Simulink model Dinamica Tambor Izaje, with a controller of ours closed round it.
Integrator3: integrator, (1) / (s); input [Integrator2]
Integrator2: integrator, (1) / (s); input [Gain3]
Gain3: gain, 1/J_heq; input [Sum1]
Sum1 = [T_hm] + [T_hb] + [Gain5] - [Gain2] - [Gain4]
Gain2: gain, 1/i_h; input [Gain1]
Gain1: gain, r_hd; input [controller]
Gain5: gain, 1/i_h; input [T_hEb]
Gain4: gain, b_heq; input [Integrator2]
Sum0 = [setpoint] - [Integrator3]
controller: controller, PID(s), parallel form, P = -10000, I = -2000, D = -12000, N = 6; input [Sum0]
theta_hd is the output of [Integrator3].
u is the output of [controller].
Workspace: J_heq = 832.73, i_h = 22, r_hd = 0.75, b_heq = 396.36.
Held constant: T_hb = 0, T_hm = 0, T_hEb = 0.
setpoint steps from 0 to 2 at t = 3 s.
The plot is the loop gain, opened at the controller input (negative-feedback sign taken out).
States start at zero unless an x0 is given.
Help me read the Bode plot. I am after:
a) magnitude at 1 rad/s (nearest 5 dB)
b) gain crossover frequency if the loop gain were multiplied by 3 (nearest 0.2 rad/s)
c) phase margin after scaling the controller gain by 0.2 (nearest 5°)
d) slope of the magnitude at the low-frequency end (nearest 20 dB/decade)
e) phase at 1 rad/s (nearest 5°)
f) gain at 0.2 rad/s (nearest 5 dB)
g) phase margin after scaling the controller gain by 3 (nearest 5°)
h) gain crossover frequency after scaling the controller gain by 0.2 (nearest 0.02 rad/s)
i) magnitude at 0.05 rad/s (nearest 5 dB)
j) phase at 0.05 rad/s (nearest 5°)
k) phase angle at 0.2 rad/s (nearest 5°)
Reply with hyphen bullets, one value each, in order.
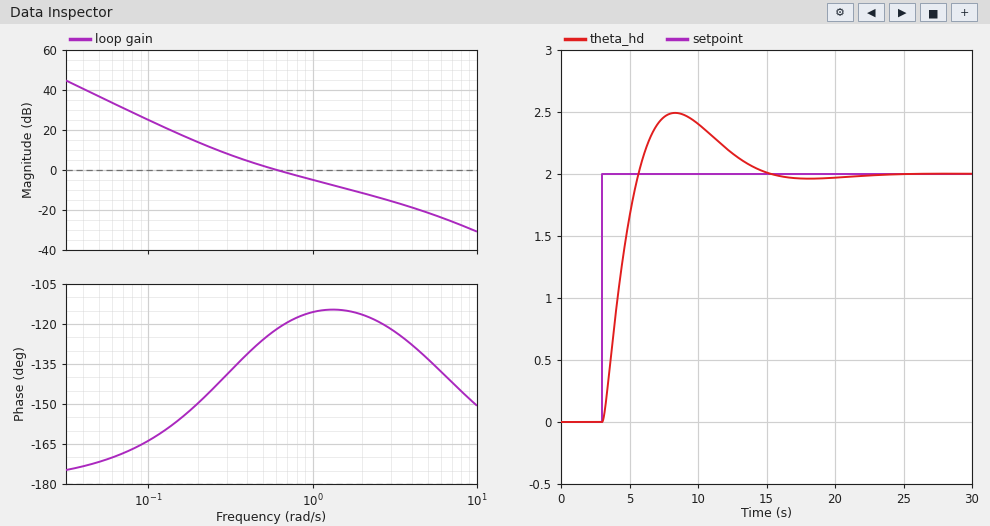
- -5 dB
- 1.6 rad/s
- 30°
- -40 dB/decade
- -115°
- 15 dB
- 65°
- 0.20 rad/s
- 35 dB
- -170°
- -150°
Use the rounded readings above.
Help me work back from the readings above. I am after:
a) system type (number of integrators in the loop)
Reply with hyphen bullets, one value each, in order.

- 2
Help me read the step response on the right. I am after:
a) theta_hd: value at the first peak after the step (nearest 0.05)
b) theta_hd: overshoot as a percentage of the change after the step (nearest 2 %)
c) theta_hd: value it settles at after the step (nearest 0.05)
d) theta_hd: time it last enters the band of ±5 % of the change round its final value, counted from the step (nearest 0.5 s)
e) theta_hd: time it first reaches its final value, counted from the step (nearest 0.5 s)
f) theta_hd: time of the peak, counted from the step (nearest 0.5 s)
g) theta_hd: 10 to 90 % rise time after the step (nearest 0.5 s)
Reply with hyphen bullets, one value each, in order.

- 2.50
- 24 %
- 2.00
- 10.5 s
- 2.5 s
- 5.5 s
- 2.0 s
